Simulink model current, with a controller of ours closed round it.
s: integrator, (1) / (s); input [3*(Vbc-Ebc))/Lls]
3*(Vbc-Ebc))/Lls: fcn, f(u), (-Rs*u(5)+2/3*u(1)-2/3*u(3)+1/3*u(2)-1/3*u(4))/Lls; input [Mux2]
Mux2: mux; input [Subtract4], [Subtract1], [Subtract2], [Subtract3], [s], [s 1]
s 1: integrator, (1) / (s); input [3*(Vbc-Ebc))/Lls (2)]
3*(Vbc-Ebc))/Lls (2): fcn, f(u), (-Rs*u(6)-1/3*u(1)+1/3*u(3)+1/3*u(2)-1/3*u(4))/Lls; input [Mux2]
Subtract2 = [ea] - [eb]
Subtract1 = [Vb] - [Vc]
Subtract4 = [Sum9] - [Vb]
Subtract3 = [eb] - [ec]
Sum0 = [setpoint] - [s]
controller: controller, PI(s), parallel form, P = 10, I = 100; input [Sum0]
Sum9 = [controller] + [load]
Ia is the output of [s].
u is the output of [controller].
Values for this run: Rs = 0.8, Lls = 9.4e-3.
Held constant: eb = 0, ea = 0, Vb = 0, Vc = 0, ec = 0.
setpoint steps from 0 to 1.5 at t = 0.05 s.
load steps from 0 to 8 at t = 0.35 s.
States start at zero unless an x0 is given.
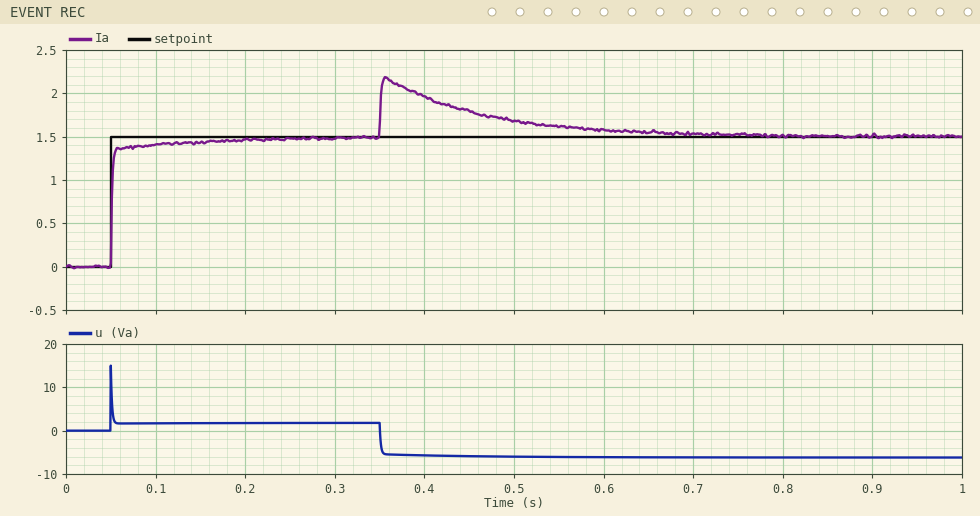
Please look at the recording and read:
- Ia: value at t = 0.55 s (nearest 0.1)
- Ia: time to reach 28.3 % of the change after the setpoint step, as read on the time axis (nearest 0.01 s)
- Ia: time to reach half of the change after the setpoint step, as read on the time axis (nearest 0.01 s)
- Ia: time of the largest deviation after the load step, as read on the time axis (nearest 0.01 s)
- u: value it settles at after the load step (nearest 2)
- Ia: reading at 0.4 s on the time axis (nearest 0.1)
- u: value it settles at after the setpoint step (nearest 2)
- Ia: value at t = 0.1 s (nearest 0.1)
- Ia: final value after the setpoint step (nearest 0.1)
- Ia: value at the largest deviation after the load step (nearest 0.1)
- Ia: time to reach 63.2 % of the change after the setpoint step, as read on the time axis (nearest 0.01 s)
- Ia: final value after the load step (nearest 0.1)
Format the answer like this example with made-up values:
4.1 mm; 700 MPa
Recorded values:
1.6; 0.05 s; 0.05 s; 0.36 s; -6; 2.0; 2; 1.4; 1.5; 2.2; 0.05 s; 1.5
